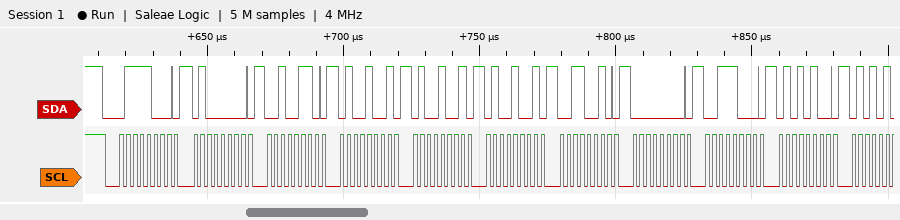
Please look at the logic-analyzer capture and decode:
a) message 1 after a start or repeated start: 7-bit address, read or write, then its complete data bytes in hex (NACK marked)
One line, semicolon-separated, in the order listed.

0x3C write: 40 26 49 49 49 32 00 38 54
